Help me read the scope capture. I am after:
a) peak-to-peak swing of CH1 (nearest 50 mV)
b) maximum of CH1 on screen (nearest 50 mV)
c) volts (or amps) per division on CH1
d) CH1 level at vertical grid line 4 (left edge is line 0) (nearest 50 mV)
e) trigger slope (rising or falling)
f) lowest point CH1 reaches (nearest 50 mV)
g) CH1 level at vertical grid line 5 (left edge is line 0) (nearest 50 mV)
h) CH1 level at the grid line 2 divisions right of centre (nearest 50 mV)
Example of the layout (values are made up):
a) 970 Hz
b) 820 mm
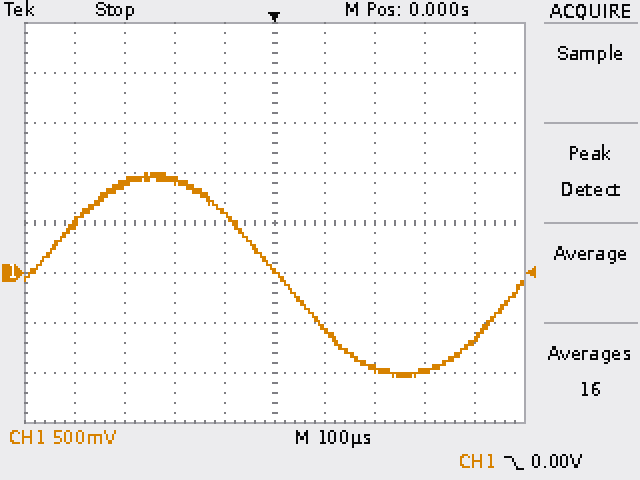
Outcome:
a) 2.05 V
b) 1.00 V
c) 500 mV
d) 600 mV
e) falling
f) -1.05 V
g) 50 mV
h) -950 mV
